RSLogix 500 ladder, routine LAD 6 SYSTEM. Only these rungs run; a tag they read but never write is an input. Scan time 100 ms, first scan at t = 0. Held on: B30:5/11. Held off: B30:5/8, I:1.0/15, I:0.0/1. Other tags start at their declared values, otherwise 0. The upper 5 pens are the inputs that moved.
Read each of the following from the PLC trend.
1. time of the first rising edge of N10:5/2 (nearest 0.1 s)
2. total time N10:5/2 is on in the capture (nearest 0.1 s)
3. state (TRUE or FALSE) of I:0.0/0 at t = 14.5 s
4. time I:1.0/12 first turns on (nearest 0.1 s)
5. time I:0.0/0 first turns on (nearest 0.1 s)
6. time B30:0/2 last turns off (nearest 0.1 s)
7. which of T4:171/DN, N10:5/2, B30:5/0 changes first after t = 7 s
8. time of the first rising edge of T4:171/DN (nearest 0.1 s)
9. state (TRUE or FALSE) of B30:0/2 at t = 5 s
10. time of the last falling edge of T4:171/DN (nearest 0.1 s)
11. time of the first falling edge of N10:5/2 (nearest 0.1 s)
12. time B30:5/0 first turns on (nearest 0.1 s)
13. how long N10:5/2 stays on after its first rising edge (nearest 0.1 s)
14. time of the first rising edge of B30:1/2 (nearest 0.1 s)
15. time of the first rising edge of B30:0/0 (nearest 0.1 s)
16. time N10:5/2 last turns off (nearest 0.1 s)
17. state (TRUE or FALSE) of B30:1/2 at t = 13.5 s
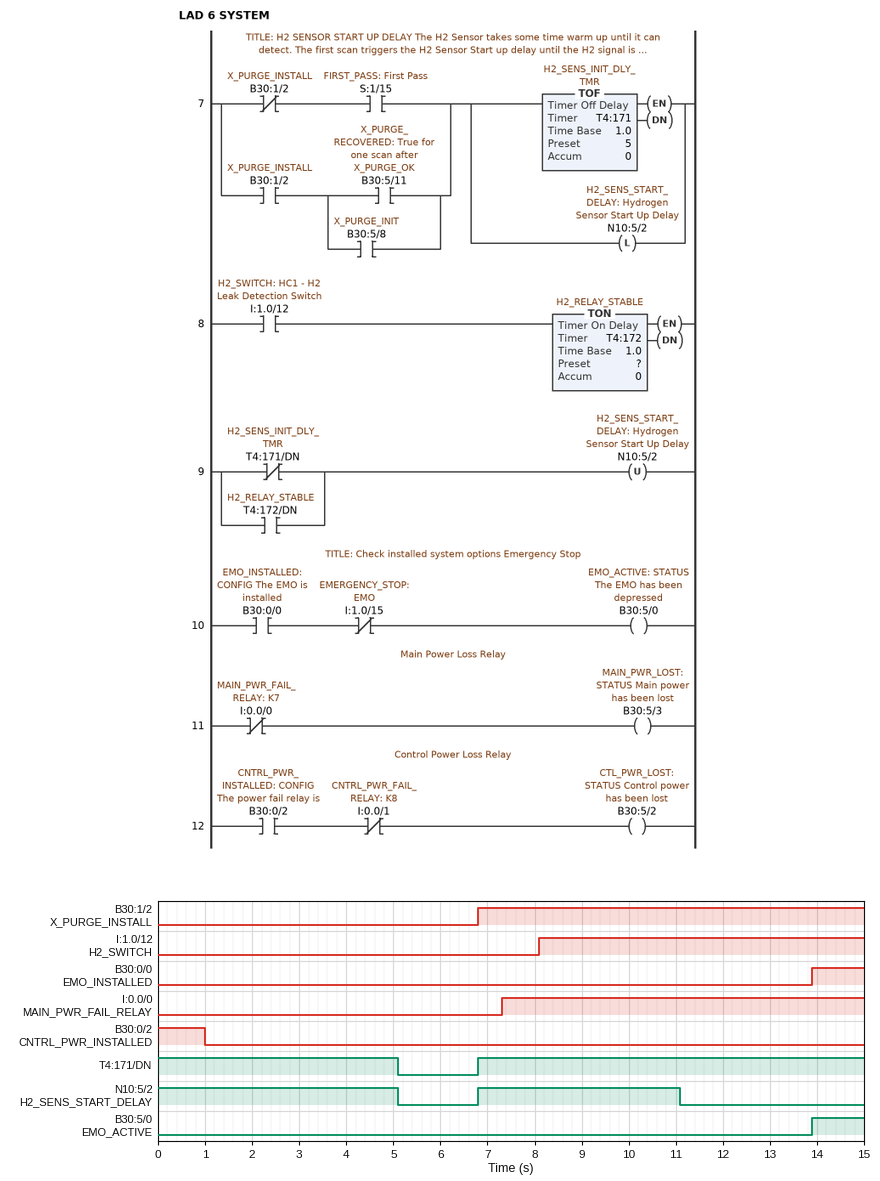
6.8 s
9.4 s
TRUE
8.1 s
7.3 s
1.0 s
N10:5/2
6.8 s
FALSE
5.1 s
5.1 s
13.9 s
4.3 s
6.8 s
13.9 s
11.1 s
TRUE
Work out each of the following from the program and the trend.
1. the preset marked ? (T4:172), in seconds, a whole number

3 s
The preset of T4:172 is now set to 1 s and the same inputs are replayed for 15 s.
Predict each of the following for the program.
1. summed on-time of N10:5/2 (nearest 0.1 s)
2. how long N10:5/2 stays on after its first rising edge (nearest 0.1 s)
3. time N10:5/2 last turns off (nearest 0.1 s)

7.4 s
2.3 s
9.1 s
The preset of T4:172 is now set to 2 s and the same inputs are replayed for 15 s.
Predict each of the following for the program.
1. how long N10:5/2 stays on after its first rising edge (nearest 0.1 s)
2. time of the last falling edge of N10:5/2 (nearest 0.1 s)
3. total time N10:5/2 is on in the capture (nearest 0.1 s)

3.3 s
10.1 s
8.4 s
